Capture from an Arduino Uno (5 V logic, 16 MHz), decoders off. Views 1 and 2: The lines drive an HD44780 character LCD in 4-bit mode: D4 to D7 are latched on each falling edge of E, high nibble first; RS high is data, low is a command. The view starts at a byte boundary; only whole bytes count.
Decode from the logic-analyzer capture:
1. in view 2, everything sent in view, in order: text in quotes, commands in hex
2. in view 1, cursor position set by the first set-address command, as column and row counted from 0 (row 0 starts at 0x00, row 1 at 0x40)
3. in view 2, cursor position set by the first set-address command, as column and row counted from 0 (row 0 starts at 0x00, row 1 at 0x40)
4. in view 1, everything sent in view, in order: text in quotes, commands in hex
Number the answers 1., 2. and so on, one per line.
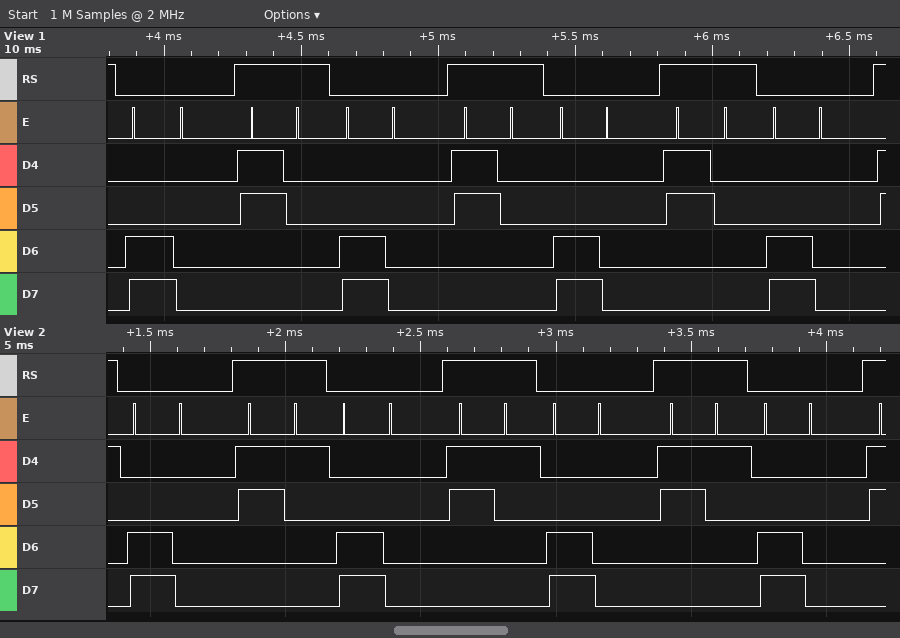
1. 0xC0 "1" 0xC0 "1" 0xC0 "1" 0xC0
2. column 0, row 1
3. column 0, row 1
4. 0xC0 "0" 0xC0 "0" 0xC0 "0" 0xC0
